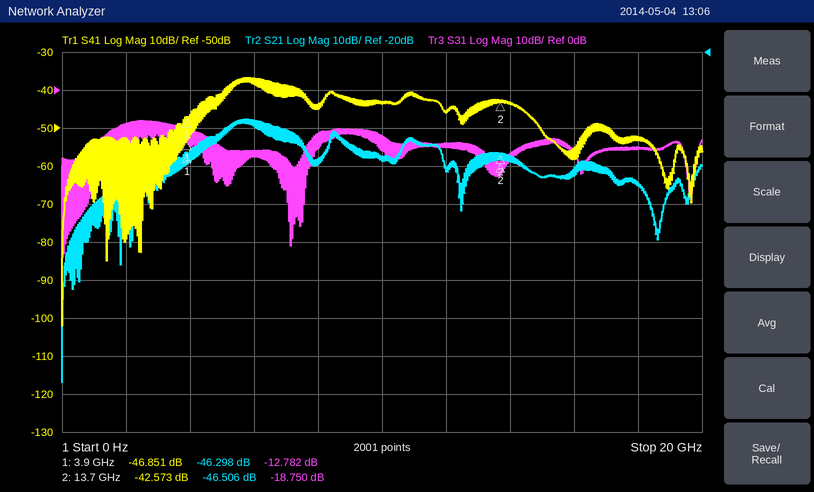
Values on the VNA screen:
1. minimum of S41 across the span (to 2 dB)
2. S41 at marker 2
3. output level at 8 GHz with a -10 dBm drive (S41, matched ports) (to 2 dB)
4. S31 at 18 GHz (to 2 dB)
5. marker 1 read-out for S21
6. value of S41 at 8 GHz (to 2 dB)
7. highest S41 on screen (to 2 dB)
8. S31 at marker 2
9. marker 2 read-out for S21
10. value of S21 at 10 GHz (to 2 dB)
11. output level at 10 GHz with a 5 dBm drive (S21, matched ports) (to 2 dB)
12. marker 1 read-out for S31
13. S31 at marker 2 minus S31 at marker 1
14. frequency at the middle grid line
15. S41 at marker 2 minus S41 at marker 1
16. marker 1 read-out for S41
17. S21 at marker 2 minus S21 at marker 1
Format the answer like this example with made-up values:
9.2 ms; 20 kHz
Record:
-102 dB; -42.573 dB; -54 dBm; -16 dB; -46.298 dB; -44 dB; -36 dB; -18.750 dB; -46.506 dB; -48 dB; -44 dBm; -12.782 dB; -5.968 dB; 10 GHz; 4.278 dB; -46.851 dB; -0.208 dB
